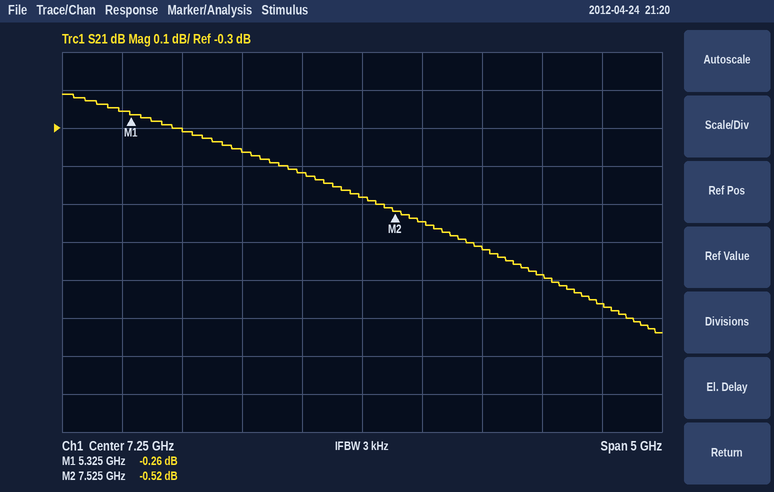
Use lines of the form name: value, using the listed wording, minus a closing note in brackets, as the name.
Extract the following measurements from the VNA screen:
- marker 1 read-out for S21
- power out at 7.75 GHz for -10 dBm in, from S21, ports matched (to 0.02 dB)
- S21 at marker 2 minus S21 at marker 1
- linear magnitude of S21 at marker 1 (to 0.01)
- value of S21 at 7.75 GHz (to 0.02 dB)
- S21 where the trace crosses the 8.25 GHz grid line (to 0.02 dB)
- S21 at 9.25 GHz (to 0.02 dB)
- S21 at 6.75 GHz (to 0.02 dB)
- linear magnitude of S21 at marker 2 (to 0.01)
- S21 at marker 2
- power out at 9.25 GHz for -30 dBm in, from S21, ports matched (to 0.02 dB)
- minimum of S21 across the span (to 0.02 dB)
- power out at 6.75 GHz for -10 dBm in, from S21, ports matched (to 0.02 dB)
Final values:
marker 1 read-out for S21: -0.26 dB
power out at 7.75 GHz for -10 dBm in, from S21, ports matched: -10.54 dBm
S21 at marker 2 minus S21 at marker 1: -0.26 dB
linear magnitude of S21 at marker 1: 0.97
value of S21 at 7.75 GHz: -0.54 dB
S21 where the trace crosses the 8.25 GHz grid line: -0.62 dB
S21 at 9.25 GHz: -0.76 dB
S21 at 6.75 GHz: -0.42 dB
linear magnitude of S21 at marker 2: 0.94
S21 at marker 2: -0.52 dB
power out at 9.25 GHz for -30 dBm in, from S21, ports matched: -30.76 dBm
minimum of S21 across the span: -0.84 dB
power out at 6.75 GHz for -10 dBm in, from S21, ports matched: -10.42 dBm
